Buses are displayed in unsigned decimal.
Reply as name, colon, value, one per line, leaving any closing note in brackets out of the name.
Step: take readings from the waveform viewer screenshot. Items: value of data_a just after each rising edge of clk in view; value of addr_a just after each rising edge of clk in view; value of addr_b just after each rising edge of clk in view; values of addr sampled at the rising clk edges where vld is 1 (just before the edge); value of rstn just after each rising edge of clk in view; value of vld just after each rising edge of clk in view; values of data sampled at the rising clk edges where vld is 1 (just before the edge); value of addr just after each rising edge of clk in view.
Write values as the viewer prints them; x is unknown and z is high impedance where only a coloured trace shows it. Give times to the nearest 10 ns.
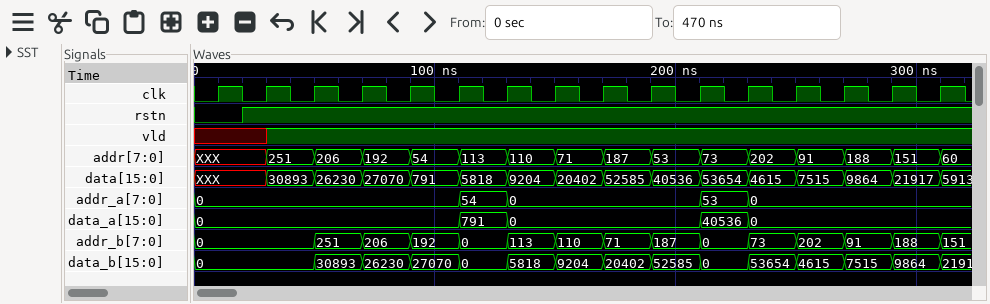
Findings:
value of data_a just after each rising edge of clk in view: 0, 0, 0, 0, 0, 791, 0, 0, 0, 0, 40536, 0, 0, 0, 0, 0
value of addr_a just after each rising edge of clk in view: 0, 0, 0, 0, 0, 54, 0, 0, 0, 0, 53, 0, 0, 0, 0, 0
value of addr_b just after each rising edge of clk in view: 0, 0, 251, 206, 192, 0, 113, 110, 71, 187, 0, 73, 202, 91, 188, 151
values of addr sampled at the rising clk edges where vld is 1: 251, 206, 192, 54, 113, 110, 71, 187, 53, 73, 202, 91, 188, 151
value of rstn just after each rising edge of clk in view: 0 1 1 1 1 1 1 1 1 1 1 1 1 1 1 1
value of vld just after each rising edge of clk in view: x 1 1 1 1 1 1 1 1 1 1 1 1 1 1 1
values of data sampled at the rising clk edges where vld is 1: 30893, 26230, 27070, 791, 5818, 9204, 20402, 52585, 40536, 53654, 4615, 7515, 9864, 21917
value of addr just after each rising edge of clk in view: XXX, 251, 206, 192, 54, 113, 110, 71, 187, 53, 73, 202, 91, 188, 151, 60
